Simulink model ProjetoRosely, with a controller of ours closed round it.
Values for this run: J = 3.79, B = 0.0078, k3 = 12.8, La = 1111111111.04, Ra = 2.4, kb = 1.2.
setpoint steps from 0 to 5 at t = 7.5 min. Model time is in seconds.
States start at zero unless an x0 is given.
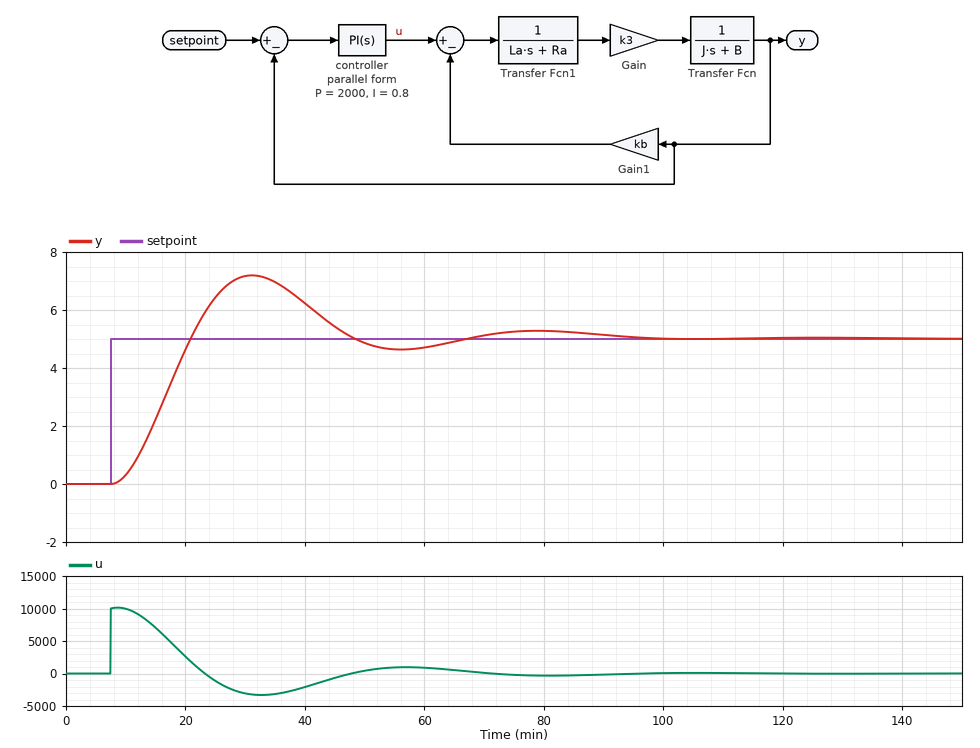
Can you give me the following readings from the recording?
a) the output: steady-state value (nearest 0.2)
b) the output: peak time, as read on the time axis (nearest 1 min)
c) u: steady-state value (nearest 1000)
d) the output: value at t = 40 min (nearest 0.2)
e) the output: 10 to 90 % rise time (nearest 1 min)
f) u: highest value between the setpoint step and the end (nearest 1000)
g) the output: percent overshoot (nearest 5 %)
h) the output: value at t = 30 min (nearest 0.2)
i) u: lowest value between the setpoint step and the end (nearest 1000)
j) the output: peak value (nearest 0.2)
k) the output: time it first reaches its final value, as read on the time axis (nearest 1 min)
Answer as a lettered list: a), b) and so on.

a) 5.0
b) 31 min
c) 0
d) 6.2
e) 9 min
f) 10000
g) 45 %
h) 7.2
i) -3000
j) 7.2
k) 21 min
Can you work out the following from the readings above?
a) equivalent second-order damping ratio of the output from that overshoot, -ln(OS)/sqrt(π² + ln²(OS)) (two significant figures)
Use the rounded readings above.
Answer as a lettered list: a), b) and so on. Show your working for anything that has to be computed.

a) ln(0.45) = -0.799; 0.799 / sqrt(9.870 + 0.638) = 0.25
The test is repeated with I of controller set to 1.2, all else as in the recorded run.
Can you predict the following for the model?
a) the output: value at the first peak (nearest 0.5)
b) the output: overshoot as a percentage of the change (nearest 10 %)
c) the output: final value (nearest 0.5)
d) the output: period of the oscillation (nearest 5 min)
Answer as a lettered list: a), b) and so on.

a) 7.5
b) 50 %
c) 5.0
d) 50 min
